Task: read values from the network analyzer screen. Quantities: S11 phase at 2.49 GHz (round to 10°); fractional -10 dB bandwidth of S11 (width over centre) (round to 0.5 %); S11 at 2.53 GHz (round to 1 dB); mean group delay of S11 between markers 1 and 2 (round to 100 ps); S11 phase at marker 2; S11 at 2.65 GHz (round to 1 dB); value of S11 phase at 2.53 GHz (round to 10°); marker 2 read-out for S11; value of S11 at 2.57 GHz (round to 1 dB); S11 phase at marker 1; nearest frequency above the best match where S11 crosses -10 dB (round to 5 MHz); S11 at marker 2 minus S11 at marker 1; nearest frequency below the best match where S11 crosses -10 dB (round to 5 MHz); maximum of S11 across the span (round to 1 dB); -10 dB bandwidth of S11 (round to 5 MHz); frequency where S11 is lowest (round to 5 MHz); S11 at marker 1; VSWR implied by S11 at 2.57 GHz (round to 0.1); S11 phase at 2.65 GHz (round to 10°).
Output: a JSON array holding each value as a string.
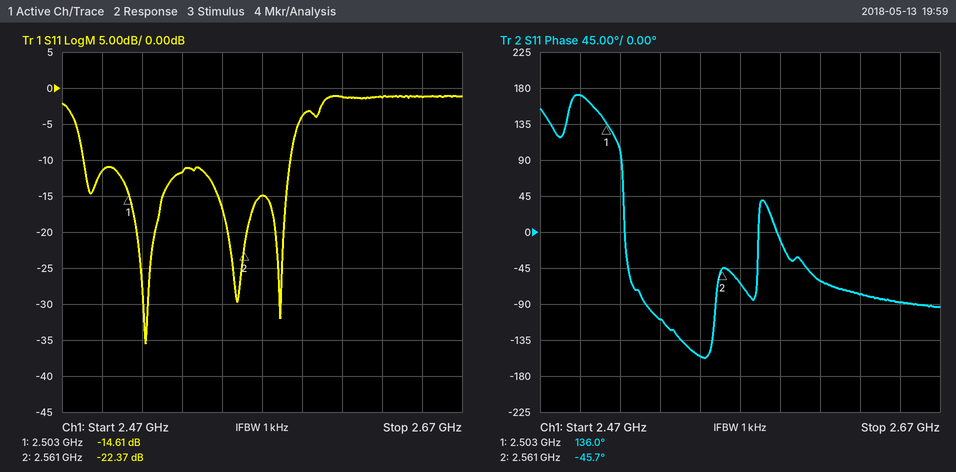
["170°", "4.0 %", "-12 dB", "8.7 ns", "-45.7°", "-1 dB", "-110°", "-22.37 dB", "-15 dB", "136.0°", "2.585 GHz", "-7.76 dB", "2.480 GHz", "-1 dB", "105 MHz", "2.510 GHz", "-14.61 dB", "1.4", "-90°"]
